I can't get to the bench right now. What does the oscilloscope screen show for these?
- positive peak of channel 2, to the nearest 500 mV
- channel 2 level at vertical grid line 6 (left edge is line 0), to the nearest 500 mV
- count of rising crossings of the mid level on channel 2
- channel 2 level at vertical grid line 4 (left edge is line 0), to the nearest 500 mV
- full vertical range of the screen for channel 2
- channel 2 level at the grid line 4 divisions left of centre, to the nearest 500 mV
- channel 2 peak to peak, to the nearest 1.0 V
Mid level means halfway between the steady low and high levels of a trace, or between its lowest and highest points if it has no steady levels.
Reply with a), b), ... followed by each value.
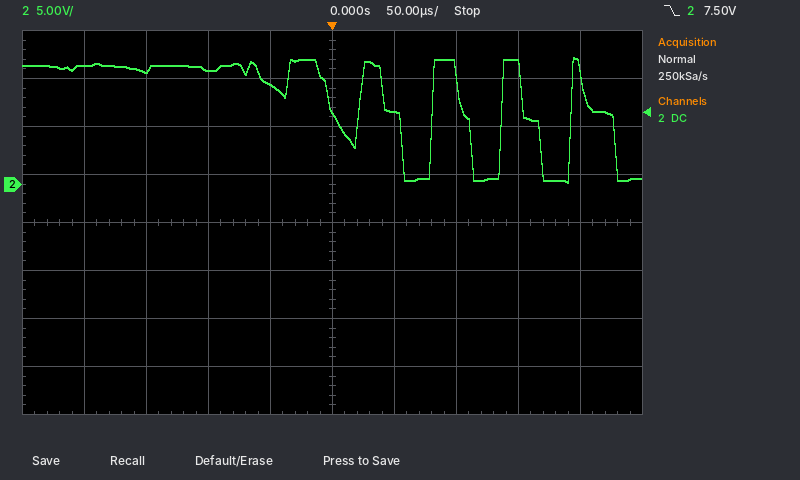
a) 13.0 V
b) 7.5 V
c) 4
d) 10.5 V
e) 40 V
f) 12.5 V
g) 13.0 V
